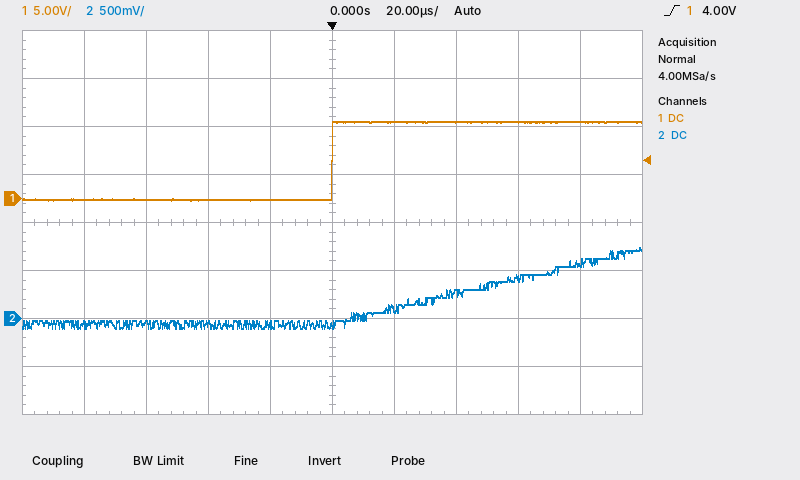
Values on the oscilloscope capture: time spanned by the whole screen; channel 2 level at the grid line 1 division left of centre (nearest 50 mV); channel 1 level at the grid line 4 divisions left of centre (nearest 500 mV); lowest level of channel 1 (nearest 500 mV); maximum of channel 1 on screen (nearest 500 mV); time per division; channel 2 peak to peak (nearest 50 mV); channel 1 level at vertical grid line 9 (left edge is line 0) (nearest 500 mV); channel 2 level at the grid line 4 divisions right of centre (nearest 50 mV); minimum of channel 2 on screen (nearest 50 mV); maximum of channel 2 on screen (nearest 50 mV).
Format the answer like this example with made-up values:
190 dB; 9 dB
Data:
200 µs; -50 mV; 0.0 V; 0.0 V; 8.0 V; 20 µs; 850 mV; 8.0 V; 600 mV; -100 mV; 750 mV
